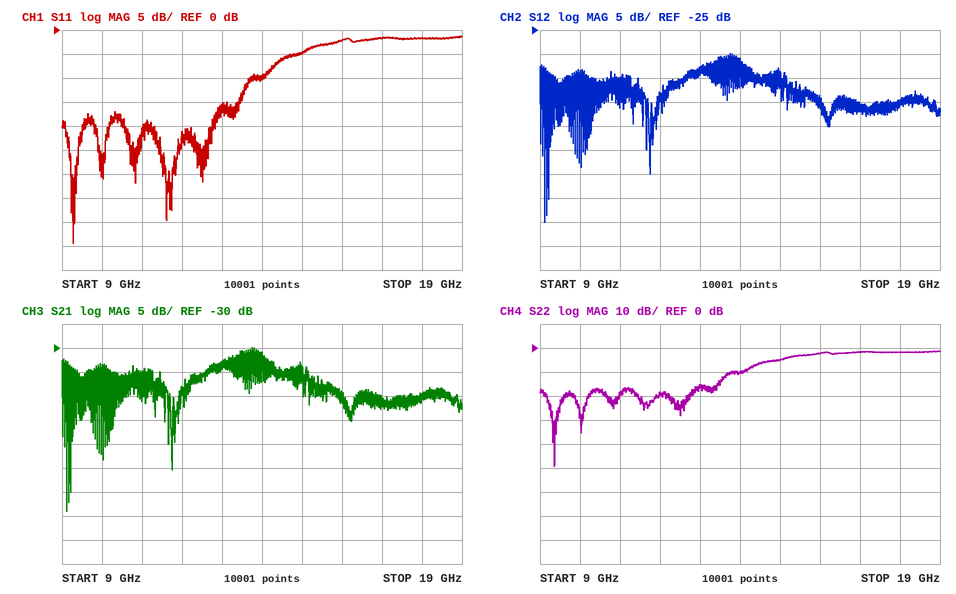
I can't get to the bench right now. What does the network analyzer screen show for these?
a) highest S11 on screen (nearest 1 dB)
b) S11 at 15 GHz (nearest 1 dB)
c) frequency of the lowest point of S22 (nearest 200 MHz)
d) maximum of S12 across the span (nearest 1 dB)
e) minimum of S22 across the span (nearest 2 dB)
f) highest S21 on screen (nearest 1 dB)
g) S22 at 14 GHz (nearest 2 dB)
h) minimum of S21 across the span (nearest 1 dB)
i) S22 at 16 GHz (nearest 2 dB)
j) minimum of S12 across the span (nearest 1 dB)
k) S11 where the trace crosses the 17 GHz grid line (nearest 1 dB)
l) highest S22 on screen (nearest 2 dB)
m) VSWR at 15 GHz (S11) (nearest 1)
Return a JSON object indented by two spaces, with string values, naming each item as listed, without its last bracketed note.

{
  "highest S11 on screen": "-1 dB",
  "S11 at 15 GHz": "-5 dB",
  "frequency of the lowest point of S22": "9.4 GHz",
  "maximum of S12 across the span": "-30 dB",
  "minimum of S22 across the span": "-50 dB",
  "highest S21 on screen": "-30 dB",
  "S22 at 14 GHz": "-10 dB",
  "minimum of S21 across the span": "-64 dB",
  "S22 at 16 GHz": "-2 dB",
  "minimum of S12 across the span": "-65 dB",
  "S11 where the trace crosses the 17 GHz grid line": "-2 dB",
  "highest S22 on screen": "-2 dB",
  "VSWR at 15 GHz (S11)": "4"
}
